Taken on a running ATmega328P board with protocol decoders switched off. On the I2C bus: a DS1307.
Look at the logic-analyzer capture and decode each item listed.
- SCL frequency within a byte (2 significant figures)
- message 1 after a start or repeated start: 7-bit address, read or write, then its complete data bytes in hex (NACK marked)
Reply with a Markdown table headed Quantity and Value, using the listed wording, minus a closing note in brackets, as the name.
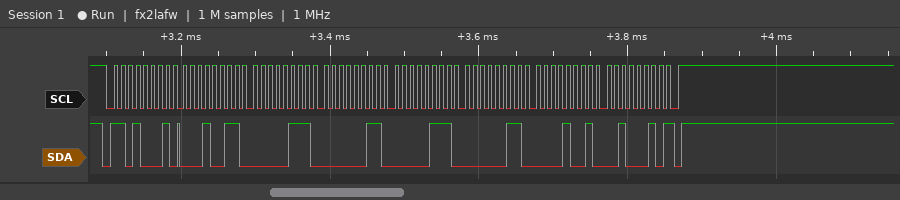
| Quantity | Value |
|---|---|
| SCL frequency within a byte | 100 kHz |
| message 1 after a start or repeated start: 7-bit address, read or write, then its complete data bytes in hex | 0x68 read: 13 07 03 07 03 09 22 NACK |
